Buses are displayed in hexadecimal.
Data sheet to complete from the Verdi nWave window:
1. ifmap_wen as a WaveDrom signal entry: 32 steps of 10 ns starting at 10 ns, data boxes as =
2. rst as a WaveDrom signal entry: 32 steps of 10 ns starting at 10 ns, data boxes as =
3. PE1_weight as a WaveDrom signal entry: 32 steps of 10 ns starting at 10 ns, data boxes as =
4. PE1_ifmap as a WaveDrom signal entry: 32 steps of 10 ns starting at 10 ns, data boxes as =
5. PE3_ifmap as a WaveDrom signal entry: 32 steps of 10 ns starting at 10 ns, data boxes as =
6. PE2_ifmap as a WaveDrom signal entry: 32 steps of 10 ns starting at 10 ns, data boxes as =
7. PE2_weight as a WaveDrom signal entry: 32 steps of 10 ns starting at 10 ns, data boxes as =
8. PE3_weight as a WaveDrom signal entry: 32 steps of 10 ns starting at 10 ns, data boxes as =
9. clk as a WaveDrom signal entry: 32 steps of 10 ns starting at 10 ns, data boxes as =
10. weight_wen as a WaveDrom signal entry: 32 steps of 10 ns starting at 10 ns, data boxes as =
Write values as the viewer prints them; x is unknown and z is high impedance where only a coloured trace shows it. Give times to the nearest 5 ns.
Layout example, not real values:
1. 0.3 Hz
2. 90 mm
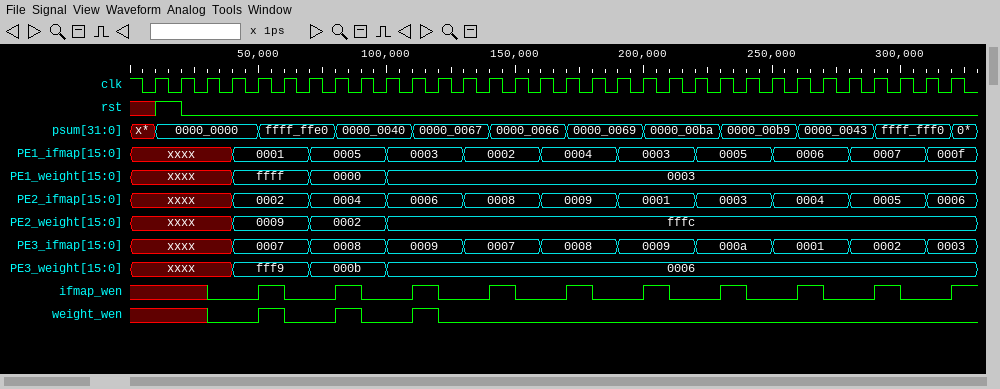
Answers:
1. {name: 'ifmap_wen', wave: 'x.0.10.10.10.10.10.10.10.10.10.1'}
2. {name: 'rst', wave: '10..............................'}
3. {name: 'PE1_weight', wave: 'x..=..=..=......................', data: 'ffff 0000 0003'}
4. {name: 'PE1_ifmap', wave: 'x..=..=..=..=..=..=..=..=..=..=.', data: '0001 0005 0003 0002 0004 0003 0005 0006 0007 000f'}
5. {name: 'PE3_ifmap', wave: 'x..=..=..=..=..=..=..=..=..=..=.', data: '0007 0008 0009 0007 0008 0009 000a 0001 0002 0003'}
6. {name: 'PE2_ifmap', wave: 'x..=..=..=..=..=..=..=..=..=..=.', data: '0002 0004 0006 0008 0009 0001 0003 0004 0005 0006'}
7. {name: 'PE2_weight', wave: 'x..=..=..=......................', data: '0009 0002 fffc'}
8. {name: 'PE3_weight', wave: 'x..=..=..=......................', data: 'fff9 000b 0006'}
9. {name: 'clk', wave: 'p...............................'}
10. {name: 'weight_wen', wave: 'x.0.10.10.10....................'}
